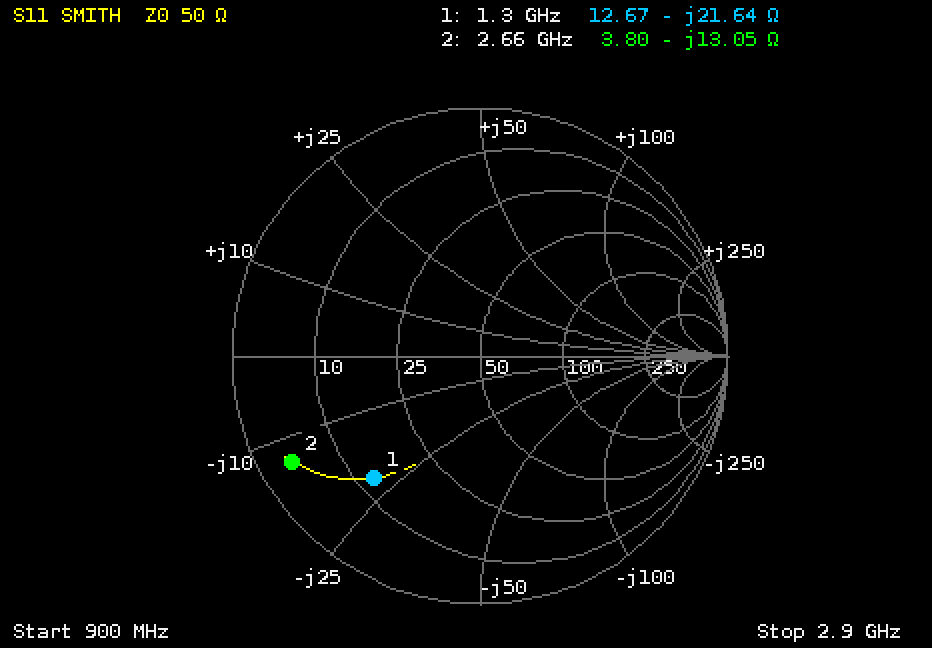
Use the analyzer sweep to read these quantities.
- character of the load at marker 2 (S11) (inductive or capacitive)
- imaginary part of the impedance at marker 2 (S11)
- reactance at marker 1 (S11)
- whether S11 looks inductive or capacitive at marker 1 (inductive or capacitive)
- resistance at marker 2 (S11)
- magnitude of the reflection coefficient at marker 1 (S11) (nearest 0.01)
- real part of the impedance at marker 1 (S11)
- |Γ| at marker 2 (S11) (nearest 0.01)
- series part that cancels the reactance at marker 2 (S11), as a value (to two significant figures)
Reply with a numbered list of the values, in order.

1. capacitive
2. -13.05 Ω
3. -21.64 Ω
4. capacitive
5. 3.80 Ω
6. 0.65
7. 12.67 Ω
8. 0.87
9. 780 pH
